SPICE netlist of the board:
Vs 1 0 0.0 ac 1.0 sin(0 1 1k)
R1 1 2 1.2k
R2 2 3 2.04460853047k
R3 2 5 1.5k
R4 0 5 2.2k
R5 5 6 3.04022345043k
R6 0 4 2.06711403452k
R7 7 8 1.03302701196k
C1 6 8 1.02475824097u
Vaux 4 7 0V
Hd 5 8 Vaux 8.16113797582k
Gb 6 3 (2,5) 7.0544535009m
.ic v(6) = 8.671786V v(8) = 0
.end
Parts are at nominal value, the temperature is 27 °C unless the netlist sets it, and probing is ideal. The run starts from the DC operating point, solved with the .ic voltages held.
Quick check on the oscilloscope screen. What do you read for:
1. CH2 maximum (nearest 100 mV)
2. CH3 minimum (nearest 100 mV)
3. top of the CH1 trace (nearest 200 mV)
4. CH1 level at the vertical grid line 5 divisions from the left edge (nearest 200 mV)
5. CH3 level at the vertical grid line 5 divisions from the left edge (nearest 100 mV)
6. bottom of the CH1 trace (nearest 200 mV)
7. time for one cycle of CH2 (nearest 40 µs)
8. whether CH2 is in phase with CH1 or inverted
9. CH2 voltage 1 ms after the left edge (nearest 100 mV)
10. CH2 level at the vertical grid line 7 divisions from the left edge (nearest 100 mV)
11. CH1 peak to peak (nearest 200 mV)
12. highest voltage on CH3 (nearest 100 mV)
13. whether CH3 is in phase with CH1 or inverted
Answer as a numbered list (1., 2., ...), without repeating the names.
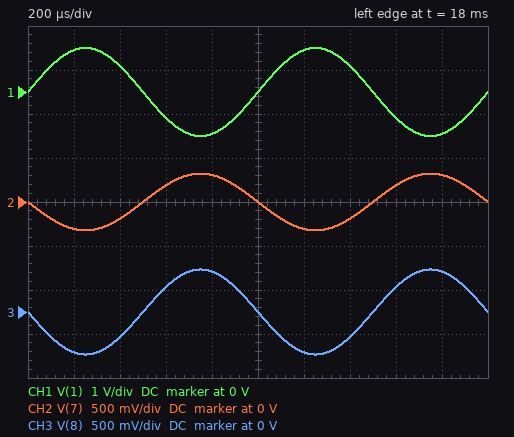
1. 300 mV
2. -500 mV
3. 1.0 V
4. 0 V
5. 0 V
6. -1.0 V
7. 1.00 ms
8. inverted
9. 0 V
10. -200 mV
11. 2.0 V
12. 500 mV
13. inverted
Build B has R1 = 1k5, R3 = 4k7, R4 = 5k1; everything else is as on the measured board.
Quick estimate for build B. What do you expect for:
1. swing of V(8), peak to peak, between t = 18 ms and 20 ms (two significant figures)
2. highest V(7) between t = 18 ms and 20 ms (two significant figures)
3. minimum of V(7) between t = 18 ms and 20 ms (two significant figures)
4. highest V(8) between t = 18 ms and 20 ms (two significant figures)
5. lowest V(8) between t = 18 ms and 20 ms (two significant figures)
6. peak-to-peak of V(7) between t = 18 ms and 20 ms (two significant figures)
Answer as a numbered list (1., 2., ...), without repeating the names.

1. 1.2 V
2. 410 mV
3. -410 mV
4. 610 mV
5. -610 mV
6. 820 mV
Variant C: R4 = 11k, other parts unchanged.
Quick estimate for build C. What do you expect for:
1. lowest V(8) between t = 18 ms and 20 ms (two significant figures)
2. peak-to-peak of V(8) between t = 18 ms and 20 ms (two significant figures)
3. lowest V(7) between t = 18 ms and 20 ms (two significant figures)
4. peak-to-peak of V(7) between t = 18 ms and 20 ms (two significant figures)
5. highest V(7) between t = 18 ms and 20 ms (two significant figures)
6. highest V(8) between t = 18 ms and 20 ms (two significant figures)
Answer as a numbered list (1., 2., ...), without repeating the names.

1. -690 mV
2. 1.4 V
3. -460 mV
4. 920 mV
5. 460 mV
6. 690 mV
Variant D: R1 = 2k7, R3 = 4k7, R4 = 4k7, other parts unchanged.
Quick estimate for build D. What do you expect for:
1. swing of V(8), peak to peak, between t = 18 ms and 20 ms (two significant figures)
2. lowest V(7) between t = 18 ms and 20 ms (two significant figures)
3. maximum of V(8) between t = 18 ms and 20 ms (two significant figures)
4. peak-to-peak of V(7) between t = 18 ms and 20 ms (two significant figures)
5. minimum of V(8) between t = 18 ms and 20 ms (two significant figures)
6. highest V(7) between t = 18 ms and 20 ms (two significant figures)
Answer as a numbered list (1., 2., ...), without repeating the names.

1. 1.2 V
2. -390 mV
3. 590 mV
4. 790 mV
5. -590 mV
6. 390 mV
